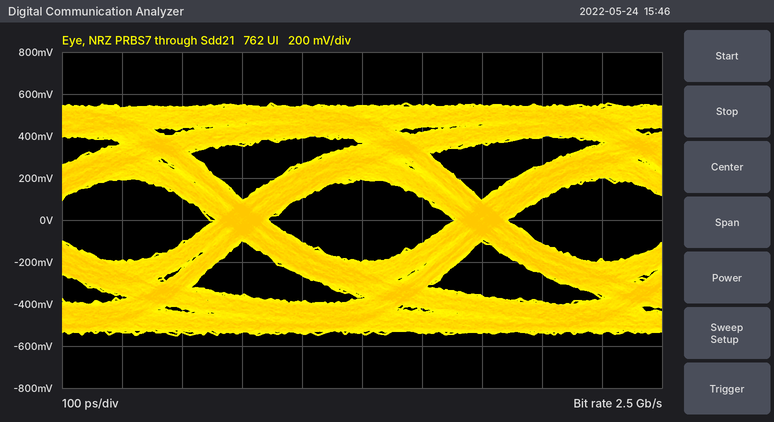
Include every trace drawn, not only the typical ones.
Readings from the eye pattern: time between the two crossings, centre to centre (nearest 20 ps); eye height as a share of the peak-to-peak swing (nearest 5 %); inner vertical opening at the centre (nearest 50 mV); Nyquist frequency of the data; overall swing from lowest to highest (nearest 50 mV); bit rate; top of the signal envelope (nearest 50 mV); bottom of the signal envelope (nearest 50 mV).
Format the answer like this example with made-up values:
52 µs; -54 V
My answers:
400 ps; 35 %; 400 mV; 1.25 GHz; 1.10 V; 2.5 Gb/s; 550 mV; -550 mV
